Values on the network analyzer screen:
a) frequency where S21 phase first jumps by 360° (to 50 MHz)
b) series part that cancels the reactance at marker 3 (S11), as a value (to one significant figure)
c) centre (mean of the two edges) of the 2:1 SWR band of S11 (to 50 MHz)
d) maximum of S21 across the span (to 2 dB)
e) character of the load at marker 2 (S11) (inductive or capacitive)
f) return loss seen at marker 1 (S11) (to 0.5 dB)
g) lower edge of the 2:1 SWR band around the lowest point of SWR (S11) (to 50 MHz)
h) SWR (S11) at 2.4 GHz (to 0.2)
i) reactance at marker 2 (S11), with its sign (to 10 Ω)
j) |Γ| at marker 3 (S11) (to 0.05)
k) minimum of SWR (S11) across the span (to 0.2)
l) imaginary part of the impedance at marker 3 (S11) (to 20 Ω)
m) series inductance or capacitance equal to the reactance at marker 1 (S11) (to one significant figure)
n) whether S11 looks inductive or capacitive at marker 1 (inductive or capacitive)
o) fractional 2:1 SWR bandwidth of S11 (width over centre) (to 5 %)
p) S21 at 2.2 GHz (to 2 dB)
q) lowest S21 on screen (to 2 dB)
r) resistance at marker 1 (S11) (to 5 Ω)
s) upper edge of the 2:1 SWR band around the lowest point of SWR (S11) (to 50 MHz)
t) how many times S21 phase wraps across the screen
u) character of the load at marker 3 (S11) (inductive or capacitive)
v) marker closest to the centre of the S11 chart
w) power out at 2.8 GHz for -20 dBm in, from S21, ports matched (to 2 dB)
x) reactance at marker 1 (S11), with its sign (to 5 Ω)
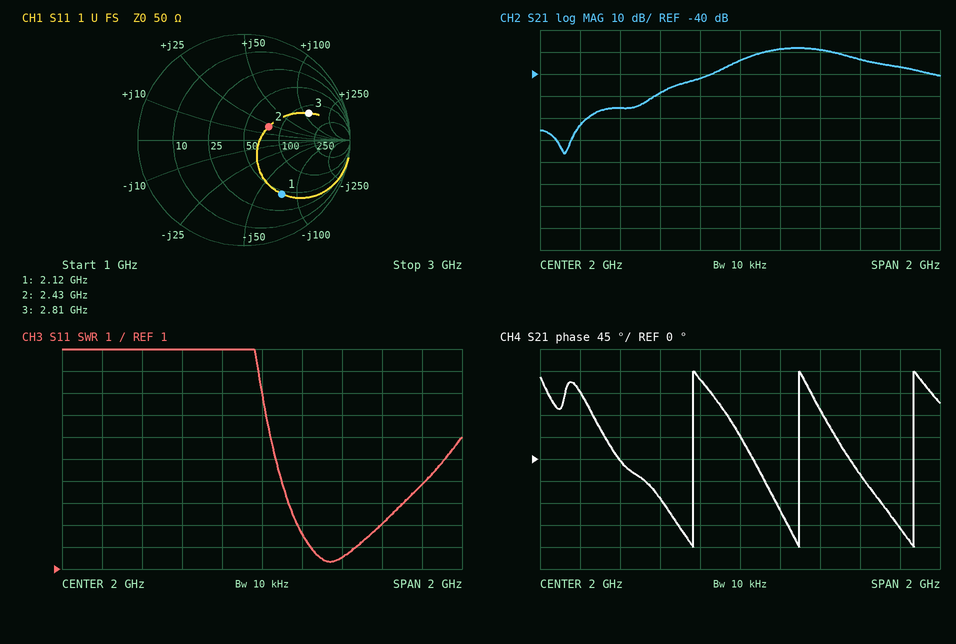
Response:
1.75 GHz
500 fF
2.35 GHz
-28 dB
inductive
4.0 dB
2.25 GHz
1.6
+20 Ω
0.65
1.4
+120 Ω
1.0 pF
capacitive
10 %
-28 dB
-76 dB
45 Ω
2.45 GHz
3
inductive
marker 2
-56 dBm
-75 Ω
